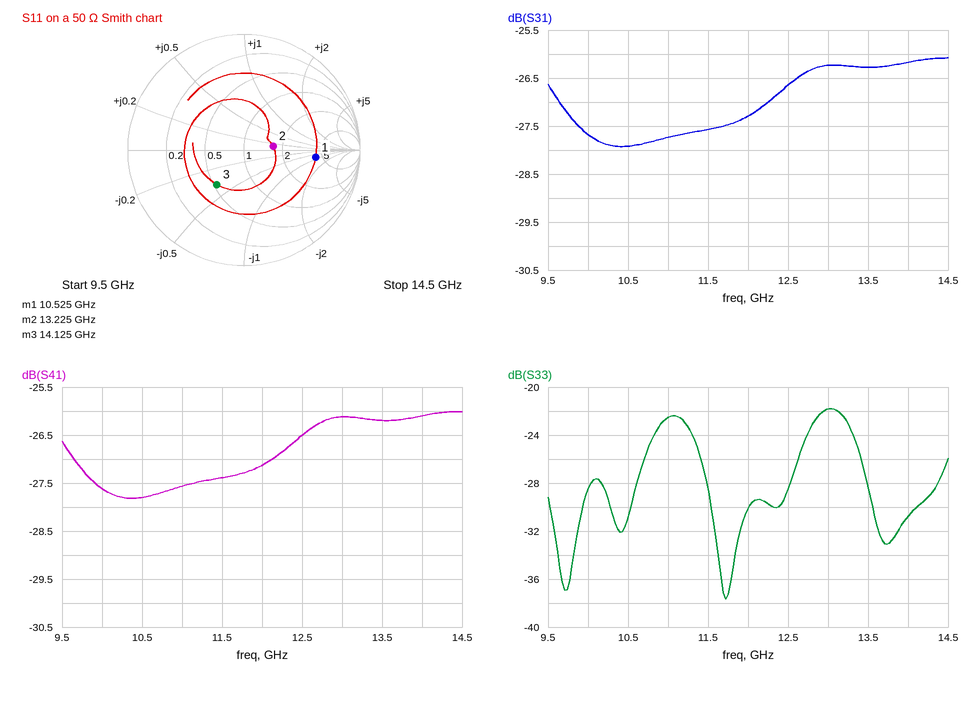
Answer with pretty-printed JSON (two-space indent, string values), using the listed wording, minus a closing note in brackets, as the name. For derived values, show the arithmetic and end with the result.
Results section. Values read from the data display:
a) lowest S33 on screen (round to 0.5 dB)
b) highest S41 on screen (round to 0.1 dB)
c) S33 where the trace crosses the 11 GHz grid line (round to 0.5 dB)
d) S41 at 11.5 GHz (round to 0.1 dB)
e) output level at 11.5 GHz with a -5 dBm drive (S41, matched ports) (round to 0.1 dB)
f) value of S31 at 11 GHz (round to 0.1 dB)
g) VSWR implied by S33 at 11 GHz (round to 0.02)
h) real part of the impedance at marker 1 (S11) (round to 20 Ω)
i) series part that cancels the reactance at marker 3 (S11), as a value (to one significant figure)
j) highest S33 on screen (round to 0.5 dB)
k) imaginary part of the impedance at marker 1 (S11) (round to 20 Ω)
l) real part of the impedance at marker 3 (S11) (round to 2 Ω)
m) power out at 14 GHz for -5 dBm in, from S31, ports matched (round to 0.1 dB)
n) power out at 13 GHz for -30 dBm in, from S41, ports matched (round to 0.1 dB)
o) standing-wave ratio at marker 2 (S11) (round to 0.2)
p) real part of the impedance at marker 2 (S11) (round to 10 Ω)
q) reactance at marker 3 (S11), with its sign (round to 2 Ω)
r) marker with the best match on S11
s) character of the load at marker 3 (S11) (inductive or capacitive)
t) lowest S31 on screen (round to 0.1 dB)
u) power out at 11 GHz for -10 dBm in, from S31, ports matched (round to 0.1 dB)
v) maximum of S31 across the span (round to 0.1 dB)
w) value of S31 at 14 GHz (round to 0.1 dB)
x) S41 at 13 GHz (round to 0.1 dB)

{
  "lowest S33 on screen": "-37.5 dB",
  "highest S41 on screen": "-26.0 dB",
  "S33 where the trace crosses the 11 GHz grid line": "-22.5 dB",
  "S41 at 11.5 GHz": "-27.4 dB",
  "output level at 11.5 GHz with a -5 dBm drive (S41, matched ports)": "-5 dBm + (-27.4 dB) = -32.4 dBm",
  "value of S31 at 11 GHz": "-27.7 dB",
  "VSWR implied by S33 at 11 GHz": "|Γ| = 10^(-22.5/20) = 0.0750; VSWR = (1 + 0.0750)/(1 − 0.0750) ≈ 1.16",
  "real part of the impedance at marker 1 (S11)": "200 Ω",
  "series part that cancels the reactance at marker 3 (S11), as a value": "L = 18 Ω/(2π × 14.125 GHz) ≈ 203 pH, so 200 pH to one significant figure",
  "highest S33 on screen": "-22.0 dB",
  "imaginary part of the impedance at marker 1 (S11)": "-40 Ω",
  "real part of the impedance at marker 3 (S11)": "26 Ω",
  "power out at 14 GHz for -5 dBm in, from S31, ports matched": "-5 dBm + (-26.2 dB) = -31.2 dBm",
  "power out at 13 GHz for -30 dBm in, from S41, ports matched": "-30 dBm + (-26.1 dB) = -56.1 dBm",
  "standing-wave ratio at marker 2 (S11)": "1.6",
  "real part of the impedance at marker 2 (S11)": "80 Ω",
  "reactance at marker 3 (S11), with its sign": "-18 Ω",
  "marker with the best match on S11": "marker 2",
  "character of the load at marker 3 (S11)": "capacitive",
  "lowest S31 on screen": "-27.9 dB",
  "power out at 11 GHz for -10 dBm in, from S31, ports matched": "-10 dBm + (-27.7 dB) = -37.7 dBm",
  "maximum of S31 across the span": "-26.1 dB",
  "value of S31 at 14 GHz": "-26.2 dB",
  "S41 at 13 GHz": "-26.1 dB"
}
